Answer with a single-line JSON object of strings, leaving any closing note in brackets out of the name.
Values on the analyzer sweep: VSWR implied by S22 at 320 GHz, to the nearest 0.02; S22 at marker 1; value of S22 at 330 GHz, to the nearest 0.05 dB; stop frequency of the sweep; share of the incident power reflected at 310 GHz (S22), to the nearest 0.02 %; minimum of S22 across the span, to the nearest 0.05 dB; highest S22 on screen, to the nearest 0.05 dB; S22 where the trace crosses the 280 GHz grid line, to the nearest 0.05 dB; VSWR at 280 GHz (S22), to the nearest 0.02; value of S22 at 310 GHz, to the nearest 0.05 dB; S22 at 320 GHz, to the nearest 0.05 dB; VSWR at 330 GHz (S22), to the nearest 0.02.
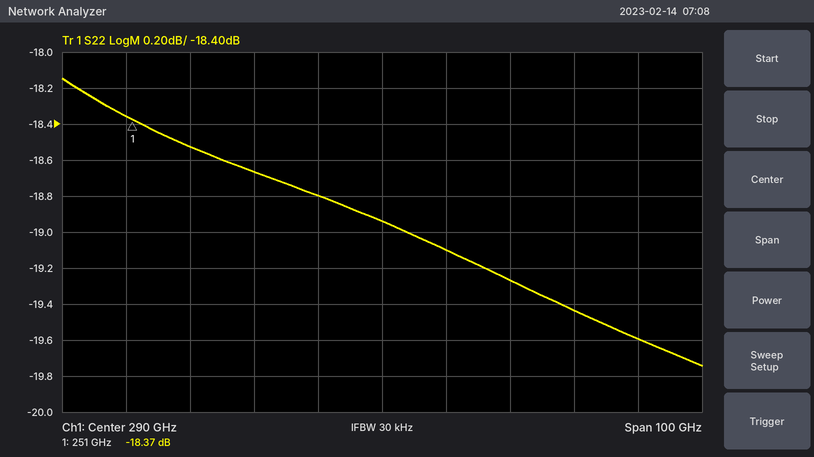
{"VSWR implied by S22 at 320 GHz, to the nearest 0.02": "1.24", "S22 at marker 1": "-18.37 dB", "value of S22 at 330 GHz, to the nearest 0.05 dB": "-19.60 dB", "stop frequency of the sweep": "340 GHz", "share of the incident power reflected at 310 GHz (S22), to the nearest 0.02 %": "1.18 %", "minimum of S22 across the span, to the nearest 0.05 dB": "-19.75 dB", "highest S22 on screen, to the nearest 0.05 dB": "-18.15 dB", "S22 where the trace crosses the 280 GHz grid line, to the nearest 0.05 dB": "-18.80 dB", "VSWR at 280 GHz (S22), to the nearest 0.02": "1.26", "value of S22 at 310 GHz, to the nearest 0.05 dB": "-19.25 dB", "S22 at 320 GHz, to the nearest 0.05 dB": "-19.45 dB", "VSWR at 330 GHz (S22), to the nearest 0.02": "1.24"}
